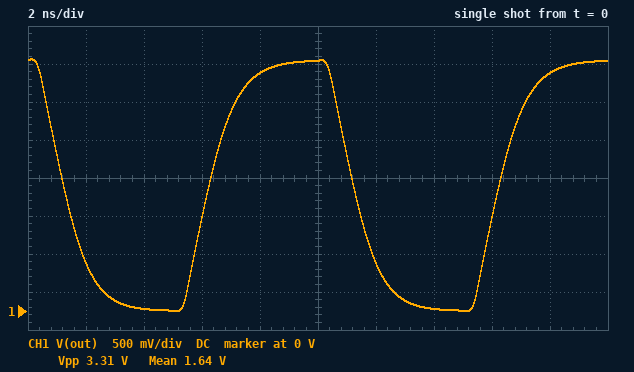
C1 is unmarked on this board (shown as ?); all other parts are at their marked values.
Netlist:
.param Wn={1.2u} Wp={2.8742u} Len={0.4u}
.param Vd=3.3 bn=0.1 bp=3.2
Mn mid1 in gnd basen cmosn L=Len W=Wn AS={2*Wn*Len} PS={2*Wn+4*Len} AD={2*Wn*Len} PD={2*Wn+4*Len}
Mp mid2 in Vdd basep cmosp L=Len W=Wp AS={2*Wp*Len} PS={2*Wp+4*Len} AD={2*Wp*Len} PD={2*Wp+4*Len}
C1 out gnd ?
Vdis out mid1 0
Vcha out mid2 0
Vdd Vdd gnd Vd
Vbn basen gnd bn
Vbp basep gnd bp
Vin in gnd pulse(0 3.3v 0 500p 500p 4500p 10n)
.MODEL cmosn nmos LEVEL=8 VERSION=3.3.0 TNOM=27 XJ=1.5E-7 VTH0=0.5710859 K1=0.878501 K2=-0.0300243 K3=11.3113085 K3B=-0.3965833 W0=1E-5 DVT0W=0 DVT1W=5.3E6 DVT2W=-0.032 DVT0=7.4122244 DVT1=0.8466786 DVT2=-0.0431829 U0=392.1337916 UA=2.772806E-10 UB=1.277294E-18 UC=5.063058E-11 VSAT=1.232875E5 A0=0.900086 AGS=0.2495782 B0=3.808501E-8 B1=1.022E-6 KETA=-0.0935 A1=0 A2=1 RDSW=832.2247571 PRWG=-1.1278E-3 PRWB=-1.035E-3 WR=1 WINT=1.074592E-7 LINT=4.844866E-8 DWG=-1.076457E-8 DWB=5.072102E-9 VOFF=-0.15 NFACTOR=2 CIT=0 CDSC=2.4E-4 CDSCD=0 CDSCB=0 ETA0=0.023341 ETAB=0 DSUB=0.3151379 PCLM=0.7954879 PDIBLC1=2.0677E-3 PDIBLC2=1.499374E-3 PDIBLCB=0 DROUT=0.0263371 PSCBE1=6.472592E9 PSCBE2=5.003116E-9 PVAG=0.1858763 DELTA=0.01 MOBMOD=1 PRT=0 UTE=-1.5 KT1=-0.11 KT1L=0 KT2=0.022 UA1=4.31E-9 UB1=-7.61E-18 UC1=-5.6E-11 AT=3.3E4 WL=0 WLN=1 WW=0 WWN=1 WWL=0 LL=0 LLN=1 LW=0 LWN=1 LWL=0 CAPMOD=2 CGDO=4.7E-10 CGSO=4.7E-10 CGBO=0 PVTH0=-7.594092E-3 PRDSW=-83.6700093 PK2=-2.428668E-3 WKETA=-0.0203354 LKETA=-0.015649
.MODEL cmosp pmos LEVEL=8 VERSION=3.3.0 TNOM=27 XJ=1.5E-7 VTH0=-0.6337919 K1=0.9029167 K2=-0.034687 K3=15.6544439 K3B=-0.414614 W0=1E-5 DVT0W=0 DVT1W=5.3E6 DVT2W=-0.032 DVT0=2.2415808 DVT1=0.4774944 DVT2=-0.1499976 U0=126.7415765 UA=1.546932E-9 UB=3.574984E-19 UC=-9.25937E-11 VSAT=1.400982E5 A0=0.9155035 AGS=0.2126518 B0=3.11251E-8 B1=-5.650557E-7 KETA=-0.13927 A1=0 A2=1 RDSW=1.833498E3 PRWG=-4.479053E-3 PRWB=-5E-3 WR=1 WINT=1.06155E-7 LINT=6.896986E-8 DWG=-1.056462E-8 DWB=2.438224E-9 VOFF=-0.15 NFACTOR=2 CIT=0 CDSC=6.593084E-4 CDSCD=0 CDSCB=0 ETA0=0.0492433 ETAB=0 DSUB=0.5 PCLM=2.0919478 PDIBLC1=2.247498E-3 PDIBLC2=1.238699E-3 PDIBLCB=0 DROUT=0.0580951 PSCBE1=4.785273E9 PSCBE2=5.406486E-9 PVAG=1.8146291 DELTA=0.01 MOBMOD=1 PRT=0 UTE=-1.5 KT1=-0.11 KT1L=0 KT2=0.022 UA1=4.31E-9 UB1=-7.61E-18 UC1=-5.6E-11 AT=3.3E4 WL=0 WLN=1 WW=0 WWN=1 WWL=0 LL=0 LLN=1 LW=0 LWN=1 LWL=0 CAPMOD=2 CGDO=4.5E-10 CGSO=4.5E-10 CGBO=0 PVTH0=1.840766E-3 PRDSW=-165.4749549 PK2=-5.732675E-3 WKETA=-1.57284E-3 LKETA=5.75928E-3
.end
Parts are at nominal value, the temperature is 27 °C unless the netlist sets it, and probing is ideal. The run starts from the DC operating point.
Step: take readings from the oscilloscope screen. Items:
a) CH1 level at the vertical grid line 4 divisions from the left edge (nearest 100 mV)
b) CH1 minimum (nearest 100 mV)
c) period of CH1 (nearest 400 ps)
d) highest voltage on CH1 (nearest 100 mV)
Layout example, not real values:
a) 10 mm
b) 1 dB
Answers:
a) 3.1 V
b) 0 V
c) 10.0 ns
d) 3.3 V
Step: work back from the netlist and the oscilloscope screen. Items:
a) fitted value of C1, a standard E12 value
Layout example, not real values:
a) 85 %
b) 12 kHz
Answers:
a) 390 fF
